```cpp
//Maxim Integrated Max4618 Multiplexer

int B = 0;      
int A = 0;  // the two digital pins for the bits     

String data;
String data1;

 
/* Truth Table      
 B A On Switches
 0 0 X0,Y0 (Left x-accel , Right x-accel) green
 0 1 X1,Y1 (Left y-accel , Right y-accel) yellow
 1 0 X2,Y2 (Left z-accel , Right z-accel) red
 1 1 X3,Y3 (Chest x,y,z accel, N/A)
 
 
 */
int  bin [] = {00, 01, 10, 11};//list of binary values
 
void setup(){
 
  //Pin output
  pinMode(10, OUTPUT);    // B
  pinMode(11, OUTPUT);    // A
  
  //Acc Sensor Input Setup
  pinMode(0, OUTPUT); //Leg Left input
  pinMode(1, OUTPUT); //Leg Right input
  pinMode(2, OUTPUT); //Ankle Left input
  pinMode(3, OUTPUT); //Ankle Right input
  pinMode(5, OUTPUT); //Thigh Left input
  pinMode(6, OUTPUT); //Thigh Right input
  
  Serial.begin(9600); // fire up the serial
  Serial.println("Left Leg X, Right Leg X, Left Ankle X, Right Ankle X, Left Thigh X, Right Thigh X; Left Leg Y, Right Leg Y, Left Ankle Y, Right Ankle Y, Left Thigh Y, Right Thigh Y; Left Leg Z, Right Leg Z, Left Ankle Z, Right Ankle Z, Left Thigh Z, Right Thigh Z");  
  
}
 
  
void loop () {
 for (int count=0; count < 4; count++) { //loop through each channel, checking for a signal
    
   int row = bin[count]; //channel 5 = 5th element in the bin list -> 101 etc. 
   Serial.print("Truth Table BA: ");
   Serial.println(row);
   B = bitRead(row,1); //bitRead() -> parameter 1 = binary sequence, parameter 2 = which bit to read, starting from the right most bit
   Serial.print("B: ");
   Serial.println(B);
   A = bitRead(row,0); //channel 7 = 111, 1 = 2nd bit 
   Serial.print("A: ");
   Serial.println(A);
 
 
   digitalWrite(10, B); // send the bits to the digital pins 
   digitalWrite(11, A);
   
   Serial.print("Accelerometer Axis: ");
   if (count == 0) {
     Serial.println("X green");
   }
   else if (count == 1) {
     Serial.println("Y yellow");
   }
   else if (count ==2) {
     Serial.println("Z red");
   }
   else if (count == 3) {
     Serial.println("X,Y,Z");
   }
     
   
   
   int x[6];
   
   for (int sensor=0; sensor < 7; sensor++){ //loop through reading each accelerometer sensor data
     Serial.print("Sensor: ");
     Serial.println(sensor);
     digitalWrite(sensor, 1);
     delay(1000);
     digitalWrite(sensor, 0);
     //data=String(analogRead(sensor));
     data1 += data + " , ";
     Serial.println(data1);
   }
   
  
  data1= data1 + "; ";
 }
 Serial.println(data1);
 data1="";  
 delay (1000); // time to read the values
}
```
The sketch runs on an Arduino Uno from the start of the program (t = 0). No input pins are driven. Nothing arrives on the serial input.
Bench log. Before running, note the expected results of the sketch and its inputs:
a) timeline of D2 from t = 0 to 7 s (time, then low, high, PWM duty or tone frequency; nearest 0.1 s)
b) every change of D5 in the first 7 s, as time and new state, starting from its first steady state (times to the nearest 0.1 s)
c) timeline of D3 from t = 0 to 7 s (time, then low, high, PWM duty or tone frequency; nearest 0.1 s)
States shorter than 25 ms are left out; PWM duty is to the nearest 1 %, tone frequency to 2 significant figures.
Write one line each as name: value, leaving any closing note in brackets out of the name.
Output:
timeline of D2 from t = 0 to 7 s: 0 s low; 2.3 s high; 3.3 s low
every change of D5 in the first 7 s, as time and new state, starting from its first steady state: 0 s low; 5.3 s high; 6.3 s low
timeline of D3 from t = 0 to 7 s: 0 s low; 3.3 s high; 4.3 s low
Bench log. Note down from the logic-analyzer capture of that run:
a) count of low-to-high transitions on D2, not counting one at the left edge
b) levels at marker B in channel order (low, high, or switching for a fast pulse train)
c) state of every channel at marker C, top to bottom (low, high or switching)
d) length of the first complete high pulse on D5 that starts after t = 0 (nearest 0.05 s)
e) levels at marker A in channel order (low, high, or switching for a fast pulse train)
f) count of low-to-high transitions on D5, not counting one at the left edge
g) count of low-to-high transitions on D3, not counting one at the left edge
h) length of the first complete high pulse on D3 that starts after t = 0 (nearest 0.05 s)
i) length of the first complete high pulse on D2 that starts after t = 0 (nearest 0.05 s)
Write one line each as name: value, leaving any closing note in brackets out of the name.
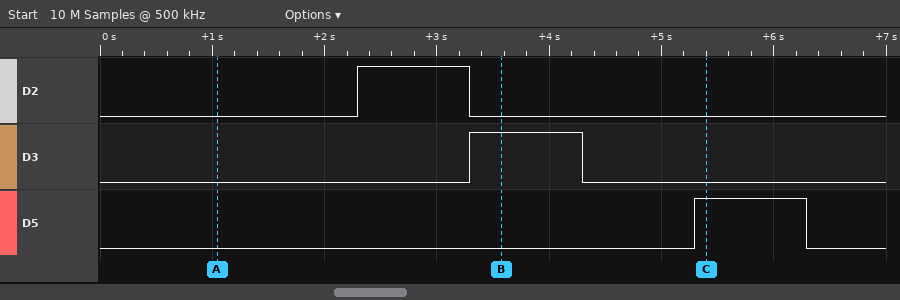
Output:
count of low-to-high transitions on D2, not counting one at the left edge: 1
levels at marker B in channel order: D2 low, D3 high, D5 low
state of every channel at marker C, top to bottom: D2 low, D3 low, D5 high
length of the first complete high pulse on D5 that starts after t = 0: 1.00 s
levels at marker A in channel order: D2 low, D3 low, D5 low
count of low-to-high transitions on D5, not counting one at the left edge: 1
count of low-to-high transitions on D3, not counting one at the left edge: 1
length of the first complete high pulse on D3 that starts after t = 0: 1.00 s
length of the first complete high pulse on D2 that starts after t = 0: 1.00 s
